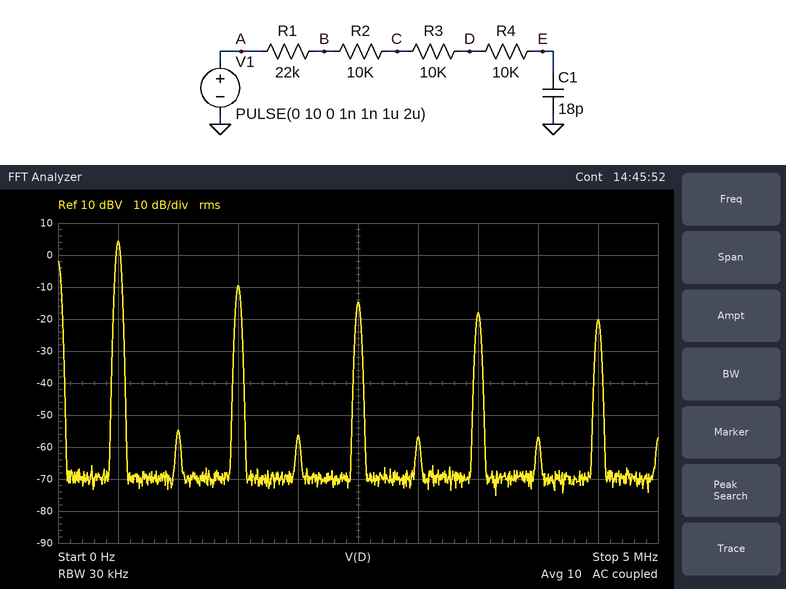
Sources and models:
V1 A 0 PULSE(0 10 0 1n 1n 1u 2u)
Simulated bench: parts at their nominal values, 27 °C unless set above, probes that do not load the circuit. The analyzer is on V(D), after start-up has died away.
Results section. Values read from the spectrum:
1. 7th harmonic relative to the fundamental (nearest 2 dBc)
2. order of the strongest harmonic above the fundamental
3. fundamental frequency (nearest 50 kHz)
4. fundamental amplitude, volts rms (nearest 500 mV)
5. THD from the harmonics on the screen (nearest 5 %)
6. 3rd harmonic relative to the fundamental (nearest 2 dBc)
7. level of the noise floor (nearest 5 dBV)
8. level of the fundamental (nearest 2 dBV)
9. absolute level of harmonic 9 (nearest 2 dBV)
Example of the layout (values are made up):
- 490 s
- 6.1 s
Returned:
- -22 dBc
- 3
- 500 kHz
- 1.5 V
- 25 %
- -14 dBc
- -70 dBV
- 4 dBV
- -20 dBV
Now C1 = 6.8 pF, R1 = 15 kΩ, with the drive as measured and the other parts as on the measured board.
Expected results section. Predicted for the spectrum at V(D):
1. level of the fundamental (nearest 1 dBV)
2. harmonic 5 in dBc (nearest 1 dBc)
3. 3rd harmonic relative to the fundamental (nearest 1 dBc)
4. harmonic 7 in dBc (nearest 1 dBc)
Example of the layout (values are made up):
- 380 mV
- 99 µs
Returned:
- 10 dBV
- -22 dBc
- -15 dBc
- -26 dBc
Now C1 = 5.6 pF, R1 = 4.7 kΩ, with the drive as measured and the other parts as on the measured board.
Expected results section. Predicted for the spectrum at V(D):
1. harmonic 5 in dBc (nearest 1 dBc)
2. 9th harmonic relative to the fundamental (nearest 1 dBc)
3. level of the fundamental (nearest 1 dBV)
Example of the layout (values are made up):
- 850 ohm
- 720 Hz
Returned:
- -20 dBc
- -27 dBc
- 12 dBV
